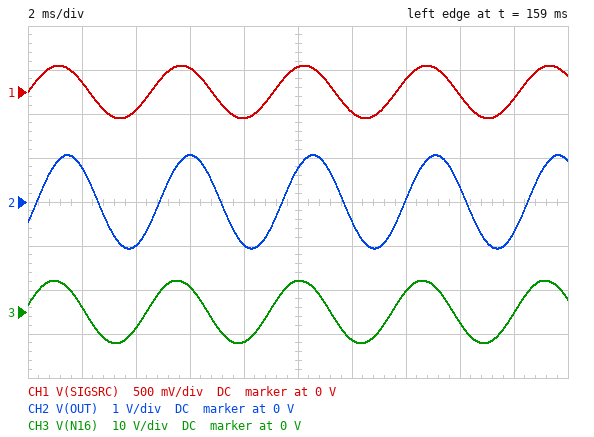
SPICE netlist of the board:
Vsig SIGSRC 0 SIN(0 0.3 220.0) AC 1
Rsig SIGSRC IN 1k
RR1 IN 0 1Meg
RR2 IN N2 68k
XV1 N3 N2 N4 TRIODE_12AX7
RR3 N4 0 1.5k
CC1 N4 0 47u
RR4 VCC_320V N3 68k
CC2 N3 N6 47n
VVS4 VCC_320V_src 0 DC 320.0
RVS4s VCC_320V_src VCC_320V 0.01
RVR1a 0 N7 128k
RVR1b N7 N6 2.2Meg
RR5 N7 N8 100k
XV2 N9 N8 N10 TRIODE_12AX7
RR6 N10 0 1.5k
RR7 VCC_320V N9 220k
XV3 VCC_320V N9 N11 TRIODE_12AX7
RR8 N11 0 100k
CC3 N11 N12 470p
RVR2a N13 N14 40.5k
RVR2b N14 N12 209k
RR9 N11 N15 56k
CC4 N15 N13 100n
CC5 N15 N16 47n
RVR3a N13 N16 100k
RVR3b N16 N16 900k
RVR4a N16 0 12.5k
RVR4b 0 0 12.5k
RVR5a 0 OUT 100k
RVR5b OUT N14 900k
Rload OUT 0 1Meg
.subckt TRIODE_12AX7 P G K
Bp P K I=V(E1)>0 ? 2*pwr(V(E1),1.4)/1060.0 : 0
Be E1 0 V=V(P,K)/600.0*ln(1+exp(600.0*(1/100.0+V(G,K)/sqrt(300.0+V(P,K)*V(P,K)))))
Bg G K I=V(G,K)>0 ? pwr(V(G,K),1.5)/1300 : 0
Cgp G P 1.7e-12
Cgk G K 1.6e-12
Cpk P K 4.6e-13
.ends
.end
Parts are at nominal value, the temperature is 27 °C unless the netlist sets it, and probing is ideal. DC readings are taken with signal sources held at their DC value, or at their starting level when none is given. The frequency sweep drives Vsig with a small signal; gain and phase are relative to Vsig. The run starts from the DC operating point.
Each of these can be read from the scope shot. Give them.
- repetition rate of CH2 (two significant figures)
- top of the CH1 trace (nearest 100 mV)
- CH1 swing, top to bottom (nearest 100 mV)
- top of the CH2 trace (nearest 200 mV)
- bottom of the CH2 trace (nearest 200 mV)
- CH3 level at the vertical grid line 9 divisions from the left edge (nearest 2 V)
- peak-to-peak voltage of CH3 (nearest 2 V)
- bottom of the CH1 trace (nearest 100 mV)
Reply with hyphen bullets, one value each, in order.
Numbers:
- 220 Hz
- 300 mV
- 600 mV
- 1.0 V
- -1.0 V
- 0 V
- 14 V
- -300 mV
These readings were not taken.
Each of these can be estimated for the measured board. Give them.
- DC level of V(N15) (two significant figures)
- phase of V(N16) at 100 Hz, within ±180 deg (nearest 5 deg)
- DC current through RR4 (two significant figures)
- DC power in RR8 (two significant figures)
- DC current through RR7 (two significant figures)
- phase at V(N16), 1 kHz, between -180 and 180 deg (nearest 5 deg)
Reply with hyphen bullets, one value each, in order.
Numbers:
- 160 V
- 25 deg
- 1.2 mA
- 250 mW
- 740 µA
- 0 deg
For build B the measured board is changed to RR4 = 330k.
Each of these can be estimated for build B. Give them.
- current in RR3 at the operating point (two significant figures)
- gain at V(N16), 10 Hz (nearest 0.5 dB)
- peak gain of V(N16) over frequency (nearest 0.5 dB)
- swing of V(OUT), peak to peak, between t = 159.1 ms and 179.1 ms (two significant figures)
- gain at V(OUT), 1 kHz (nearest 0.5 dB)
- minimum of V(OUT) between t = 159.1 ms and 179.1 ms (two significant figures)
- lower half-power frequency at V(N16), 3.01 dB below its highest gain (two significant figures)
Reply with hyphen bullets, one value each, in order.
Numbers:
- 580 µA
- 23.5 dB
- 32.0 dB
- 3.0 V
- 13.0 dB
- -1.5 V
- 79 Hz
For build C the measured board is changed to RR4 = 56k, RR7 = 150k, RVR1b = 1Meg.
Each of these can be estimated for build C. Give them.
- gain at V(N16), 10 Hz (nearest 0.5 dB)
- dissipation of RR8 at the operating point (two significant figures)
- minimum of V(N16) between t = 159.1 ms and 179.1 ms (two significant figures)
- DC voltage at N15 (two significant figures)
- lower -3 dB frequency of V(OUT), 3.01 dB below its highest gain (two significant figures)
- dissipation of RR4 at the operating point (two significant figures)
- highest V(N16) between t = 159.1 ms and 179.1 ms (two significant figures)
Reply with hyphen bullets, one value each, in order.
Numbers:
- 23.0 dB
- 350 mW
- -10 V
- 190 V
- 10 Hz
- 84 mW
- 8.6 V
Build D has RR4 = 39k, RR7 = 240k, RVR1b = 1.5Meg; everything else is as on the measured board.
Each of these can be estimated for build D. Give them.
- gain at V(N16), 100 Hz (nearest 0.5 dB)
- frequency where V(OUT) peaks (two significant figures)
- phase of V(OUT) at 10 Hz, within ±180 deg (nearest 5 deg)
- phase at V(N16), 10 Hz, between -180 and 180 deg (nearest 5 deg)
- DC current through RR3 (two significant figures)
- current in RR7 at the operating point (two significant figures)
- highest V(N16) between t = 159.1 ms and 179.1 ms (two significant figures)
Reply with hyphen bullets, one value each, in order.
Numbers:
- 27.5 dB
- 33 Hz
- 70 deg
- 75 deg
- 1.3 mA
- 700 µA
- 8.2 V
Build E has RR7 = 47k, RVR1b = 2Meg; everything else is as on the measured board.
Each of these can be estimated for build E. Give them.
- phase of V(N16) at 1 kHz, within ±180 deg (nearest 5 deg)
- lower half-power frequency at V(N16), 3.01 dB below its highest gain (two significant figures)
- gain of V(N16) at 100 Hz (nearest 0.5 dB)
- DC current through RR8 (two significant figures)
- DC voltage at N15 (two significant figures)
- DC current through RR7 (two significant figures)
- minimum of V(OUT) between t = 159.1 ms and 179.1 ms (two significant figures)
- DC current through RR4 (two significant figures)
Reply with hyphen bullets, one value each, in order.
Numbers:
- 5 deg
- 82 Hz
- 15.5 dB
- 2.5 mA
- 250 V
- 1.5 mA
- -310 mV
- 1.2 mA
